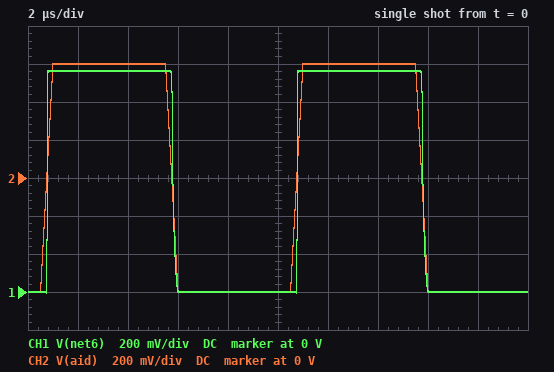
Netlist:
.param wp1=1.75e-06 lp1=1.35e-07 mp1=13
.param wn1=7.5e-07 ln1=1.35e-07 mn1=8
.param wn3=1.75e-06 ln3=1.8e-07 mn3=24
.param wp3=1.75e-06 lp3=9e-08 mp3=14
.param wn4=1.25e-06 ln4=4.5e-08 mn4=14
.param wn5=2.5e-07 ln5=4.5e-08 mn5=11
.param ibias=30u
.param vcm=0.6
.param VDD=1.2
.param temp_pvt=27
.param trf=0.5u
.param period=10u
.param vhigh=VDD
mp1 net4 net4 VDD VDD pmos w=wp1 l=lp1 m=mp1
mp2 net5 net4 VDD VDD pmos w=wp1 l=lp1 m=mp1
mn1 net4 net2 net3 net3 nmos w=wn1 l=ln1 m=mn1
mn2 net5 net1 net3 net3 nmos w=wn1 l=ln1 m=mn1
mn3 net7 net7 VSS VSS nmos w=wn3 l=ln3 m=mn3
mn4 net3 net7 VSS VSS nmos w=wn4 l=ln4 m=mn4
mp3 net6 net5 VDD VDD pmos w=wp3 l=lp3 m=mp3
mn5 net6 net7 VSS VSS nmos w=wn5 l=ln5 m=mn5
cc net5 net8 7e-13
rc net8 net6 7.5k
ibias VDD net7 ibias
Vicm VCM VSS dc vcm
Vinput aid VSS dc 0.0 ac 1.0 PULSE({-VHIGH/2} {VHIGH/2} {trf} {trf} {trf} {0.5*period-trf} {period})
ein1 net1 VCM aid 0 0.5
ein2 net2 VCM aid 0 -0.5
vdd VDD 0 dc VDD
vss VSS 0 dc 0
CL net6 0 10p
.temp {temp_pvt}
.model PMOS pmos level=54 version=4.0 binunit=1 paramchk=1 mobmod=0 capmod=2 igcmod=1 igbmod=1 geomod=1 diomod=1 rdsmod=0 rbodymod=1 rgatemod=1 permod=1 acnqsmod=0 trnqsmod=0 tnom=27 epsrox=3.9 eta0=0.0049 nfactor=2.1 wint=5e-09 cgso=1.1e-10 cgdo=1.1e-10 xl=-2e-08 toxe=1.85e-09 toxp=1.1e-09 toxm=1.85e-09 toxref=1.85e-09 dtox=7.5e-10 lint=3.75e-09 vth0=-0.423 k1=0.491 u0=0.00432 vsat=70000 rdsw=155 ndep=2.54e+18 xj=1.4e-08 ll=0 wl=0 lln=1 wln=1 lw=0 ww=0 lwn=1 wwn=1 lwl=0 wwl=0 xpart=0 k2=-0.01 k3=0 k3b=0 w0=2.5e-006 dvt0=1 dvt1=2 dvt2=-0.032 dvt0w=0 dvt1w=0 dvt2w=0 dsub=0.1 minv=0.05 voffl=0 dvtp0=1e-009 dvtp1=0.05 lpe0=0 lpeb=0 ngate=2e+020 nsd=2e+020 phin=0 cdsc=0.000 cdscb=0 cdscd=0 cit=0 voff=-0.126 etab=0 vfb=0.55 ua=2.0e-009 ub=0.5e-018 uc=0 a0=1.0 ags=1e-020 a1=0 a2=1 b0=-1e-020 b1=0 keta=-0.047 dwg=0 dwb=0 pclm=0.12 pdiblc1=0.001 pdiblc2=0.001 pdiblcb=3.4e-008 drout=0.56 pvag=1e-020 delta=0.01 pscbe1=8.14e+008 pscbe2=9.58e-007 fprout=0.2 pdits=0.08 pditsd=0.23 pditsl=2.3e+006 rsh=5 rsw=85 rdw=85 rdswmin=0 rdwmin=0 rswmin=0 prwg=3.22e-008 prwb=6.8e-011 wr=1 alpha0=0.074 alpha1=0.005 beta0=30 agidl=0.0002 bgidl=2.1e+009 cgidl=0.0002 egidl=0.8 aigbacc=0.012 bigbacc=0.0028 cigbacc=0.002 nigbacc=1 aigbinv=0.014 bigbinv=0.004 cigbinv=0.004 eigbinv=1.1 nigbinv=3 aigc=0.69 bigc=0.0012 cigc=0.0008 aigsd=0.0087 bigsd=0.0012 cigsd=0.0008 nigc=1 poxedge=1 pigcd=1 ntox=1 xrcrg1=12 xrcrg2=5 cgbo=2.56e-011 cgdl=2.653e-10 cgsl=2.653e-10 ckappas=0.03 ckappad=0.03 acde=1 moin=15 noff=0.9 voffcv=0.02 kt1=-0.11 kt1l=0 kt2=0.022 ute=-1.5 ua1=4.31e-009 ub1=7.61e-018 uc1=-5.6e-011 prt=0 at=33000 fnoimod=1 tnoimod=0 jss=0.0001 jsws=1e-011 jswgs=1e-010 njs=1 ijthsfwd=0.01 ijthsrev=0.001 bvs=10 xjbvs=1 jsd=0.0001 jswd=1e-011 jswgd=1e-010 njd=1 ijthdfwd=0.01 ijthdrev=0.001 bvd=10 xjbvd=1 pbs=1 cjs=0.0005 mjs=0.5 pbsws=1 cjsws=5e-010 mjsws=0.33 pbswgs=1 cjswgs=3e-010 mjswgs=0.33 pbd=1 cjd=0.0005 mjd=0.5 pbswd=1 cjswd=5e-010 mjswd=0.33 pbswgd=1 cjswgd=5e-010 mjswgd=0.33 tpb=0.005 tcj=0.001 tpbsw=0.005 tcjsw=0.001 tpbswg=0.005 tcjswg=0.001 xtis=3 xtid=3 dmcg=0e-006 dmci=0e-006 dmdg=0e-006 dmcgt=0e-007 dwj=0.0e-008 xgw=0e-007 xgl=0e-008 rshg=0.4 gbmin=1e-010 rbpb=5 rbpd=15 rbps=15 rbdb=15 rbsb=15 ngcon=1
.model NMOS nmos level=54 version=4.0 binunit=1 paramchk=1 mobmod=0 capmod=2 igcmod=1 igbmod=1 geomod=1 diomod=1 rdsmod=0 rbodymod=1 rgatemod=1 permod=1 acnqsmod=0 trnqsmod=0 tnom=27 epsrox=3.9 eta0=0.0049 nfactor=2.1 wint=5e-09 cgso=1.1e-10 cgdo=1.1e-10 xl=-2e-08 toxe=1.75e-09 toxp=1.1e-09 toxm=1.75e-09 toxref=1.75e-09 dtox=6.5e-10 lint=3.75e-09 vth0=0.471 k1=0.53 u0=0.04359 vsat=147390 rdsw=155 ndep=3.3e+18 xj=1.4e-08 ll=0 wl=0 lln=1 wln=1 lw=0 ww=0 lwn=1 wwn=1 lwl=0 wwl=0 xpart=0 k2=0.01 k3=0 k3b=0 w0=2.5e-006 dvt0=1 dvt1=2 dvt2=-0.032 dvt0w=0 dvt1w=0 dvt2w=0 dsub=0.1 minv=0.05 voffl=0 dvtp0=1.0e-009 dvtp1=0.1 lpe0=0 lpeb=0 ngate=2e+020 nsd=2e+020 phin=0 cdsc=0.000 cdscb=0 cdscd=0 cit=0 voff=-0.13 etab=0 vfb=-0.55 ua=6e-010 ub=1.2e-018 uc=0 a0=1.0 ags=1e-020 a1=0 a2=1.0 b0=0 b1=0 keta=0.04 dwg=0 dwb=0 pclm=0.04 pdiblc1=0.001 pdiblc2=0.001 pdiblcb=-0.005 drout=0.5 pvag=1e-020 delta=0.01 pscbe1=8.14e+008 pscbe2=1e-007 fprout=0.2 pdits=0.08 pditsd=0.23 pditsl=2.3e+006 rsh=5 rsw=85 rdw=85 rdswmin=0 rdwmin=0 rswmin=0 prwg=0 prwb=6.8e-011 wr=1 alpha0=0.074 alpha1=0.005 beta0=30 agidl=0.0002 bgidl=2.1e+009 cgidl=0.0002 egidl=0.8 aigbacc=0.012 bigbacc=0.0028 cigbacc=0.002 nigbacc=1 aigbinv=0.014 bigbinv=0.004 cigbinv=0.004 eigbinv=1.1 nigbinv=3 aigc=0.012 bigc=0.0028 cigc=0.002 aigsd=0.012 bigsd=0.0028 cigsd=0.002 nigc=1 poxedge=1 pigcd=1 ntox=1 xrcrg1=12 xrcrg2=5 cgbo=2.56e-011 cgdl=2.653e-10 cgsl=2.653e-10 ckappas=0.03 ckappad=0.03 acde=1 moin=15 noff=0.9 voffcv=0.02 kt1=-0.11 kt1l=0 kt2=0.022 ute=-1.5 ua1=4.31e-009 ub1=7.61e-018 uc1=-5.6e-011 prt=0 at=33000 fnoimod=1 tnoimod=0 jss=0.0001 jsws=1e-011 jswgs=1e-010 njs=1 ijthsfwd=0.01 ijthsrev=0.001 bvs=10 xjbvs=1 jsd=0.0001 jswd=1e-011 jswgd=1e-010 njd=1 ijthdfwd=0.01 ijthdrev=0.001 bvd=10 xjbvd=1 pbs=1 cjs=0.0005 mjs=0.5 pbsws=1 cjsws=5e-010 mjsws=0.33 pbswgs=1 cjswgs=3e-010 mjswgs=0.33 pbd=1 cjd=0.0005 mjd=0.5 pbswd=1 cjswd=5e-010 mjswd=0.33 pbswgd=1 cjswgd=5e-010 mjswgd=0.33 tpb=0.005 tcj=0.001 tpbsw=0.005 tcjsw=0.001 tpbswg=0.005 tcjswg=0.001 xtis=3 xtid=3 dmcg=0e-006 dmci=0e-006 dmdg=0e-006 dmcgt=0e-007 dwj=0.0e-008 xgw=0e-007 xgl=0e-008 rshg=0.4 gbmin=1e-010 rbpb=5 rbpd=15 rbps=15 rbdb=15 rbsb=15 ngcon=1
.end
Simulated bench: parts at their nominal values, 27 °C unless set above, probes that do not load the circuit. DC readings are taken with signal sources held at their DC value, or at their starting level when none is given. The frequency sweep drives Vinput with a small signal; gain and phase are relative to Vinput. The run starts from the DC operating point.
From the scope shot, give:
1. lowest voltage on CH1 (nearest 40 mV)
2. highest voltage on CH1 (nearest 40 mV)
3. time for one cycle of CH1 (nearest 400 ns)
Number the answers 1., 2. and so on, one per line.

1. 0 V
2. 1.16 V
3. 10.0 µs
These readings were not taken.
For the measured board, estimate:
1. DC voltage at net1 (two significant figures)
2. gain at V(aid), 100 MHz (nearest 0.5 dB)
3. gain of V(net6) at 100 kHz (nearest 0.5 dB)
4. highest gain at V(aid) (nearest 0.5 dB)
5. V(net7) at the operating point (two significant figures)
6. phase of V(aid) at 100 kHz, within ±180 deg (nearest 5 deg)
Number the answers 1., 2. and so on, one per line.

1. 600 mV
2. 0 dB
3. 49.0 dB
4. 0 dB
5. 360 mV
6. 0 deg
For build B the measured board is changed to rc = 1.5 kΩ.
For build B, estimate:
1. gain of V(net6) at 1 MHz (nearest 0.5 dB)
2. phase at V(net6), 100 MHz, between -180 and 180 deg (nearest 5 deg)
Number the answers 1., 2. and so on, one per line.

1. 44.0 dB
2. -145 deg
